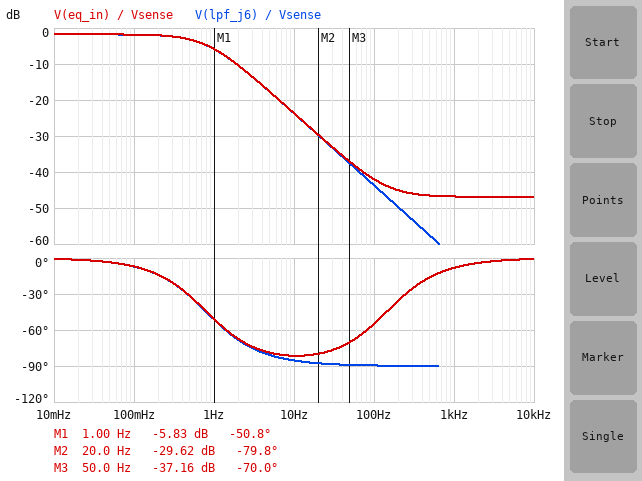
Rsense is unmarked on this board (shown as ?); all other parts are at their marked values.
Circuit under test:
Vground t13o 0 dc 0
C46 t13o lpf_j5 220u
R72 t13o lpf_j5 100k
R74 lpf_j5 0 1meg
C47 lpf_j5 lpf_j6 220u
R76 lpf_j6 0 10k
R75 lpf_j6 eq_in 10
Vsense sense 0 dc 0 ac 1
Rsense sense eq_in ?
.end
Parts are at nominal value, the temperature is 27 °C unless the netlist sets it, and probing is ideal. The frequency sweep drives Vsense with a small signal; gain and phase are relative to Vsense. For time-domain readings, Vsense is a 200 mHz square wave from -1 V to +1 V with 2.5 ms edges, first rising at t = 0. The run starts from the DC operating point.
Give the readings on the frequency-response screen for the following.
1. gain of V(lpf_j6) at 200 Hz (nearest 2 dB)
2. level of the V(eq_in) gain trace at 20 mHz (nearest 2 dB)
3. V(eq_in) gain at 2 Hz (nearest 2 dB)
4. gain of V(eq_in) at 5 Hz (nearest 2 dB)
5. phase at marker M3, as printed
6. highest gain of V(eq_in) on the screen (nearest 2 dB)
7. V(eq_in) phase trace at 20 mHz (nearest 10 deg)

-50 dB
-2 dB
-10 dB
-18 dB
-70.0 deg
-2 dB
0 deg
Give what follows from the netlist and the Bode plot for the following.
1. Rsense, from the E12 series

2.2 kΩ
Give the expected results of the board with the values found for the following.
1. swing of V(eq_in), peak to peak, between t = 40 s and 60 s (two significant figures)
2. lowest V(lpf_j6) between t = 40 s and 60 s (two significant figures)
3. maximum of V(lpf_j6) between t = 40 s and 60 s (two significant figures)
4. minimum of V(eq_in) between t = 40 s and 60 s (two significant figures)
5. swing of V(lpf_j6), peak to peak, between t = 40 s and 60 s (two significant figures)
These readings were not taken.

1.6 V
-820 mV
810 mV
-820 mV
1.6 V
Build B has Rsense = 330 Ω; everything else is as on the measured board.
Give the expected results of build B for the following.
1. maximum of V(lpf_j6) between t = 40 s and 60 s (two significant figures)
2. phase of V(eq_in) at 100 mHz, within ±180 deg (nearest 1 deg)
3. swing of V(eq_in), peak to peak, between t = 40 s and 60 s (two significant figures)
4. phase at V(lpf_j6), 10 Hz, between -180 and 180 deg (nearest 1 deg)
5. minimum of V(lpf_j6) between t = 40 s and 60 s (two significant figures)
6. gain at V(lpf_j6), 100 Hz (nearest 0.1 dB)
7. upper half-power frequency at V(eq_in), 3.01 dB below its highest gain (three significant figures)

970 mV
-1 deg
1.9 V
-66 deg
-970 mV
-27.4 dB
4.40 Hz
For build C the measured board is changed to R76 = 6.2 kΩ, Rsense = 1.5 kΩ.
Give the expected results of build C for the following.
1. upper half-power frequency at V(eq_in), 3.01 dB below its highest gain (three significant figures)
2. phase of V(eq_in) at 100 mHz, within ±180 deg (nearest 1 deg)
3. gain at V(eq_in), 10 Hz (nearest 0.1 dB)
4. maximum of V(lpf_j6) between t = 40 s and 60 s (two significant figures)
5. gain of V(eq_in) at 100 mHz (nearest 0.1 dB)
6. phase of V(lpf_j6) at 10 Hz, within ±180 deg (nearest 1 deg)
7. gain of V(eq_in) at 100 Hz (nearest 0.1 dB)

1.19 Hz
-5 deg
-20.4 dB
800 mV
-1.9 dB
-83 deg
-38.7 dB
